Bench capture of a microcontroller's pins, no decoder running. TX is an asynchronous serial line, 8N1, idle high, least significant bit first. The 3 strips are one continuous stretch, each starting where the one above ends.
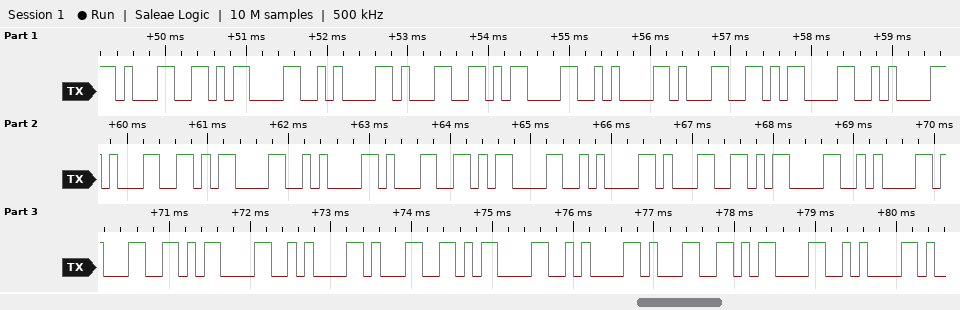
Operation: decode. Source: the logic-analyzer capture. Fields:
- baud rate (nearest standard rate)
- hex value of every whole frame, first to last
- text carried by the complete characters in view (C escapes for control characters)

9600 baud
31 0D 0A 31 0D 0A 31 0D 0A 31 0D 0A 31 0D 0A 31 0D 0A 31 0D 0A 31 0D 0A 31 0D 0A
"1\r\n1\r\n1\r\n1\r\n1\r\n1\r\n1\r\n1\r\n1\r\n"
